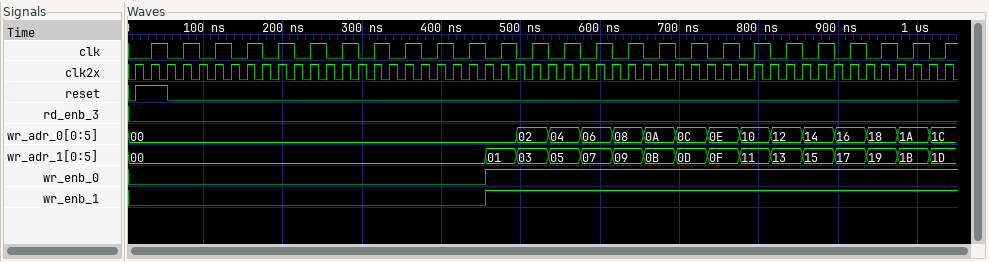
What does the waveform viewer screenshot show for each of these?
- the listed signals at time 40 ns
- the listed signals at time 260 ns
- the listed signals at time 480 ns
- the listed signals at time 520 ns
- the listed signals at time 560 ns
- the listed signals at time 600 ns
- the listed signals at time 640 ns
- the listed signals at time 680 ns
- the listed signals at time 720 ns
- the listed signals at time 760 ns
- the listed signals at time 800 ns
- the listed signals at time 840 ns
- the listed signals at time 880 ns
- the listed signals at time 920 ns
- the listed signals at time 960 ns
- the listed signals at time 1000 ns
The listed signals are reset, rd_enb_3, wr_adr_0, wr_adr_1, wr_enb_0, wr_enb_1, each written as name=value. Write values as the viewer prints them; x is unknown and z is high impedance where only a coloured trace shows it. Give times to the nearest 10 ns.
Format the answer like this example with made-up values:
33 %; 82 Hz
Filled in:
reset=1, rd_enb_3=0, wr_adr_0=00, wr_adr_1=00, wr_enb_0=0, wr_enb_1=0; reset=0, rd_enb_3=0, wr_adr_0=00, wr_adr_1=00, wr_enb_0=0, wr_enb_1=0; reset=0, rd_enb_3=0, wr_adr_0=00, wr_adr_1=01, wr_enb_0=1, wr_enb_1=1; reset=0, rd_enb_3=0, wr_adr_0=02, wr_adr_1=03, wr_enb_0=1, wr_enb_1=1; reset=0, rd_enb_3=0, wr_adr_0=04, wr_adr_1=05, wr_enb_0=1, wr_enb_1=1; reset=0, rd_enb_3=0, wr_adr_0=06, wr_adr_1=07, wr_enb_0=1, wr_enb_1=1; reset=0, rd_enb_3=0, wr_adr_0=08, wr_adr_1=09, wr_enb_0=1, wr_enb_1=1; reset=0, rd_enb_3=0, wr_adr_0=0A, wr_adr_1=0B, wr_enb_0=1, wr_enb_1=1; reset=0, rd_enb_3=0, wr_adr_0=0C, wr_adr_1=0D, wr_enb_0=1, wr_enb_1=1; reset=0, rd_enb_3=0, wr_adr_0=0E, wr_adr_1=0F, wr_enb_0=1, wr_enb_1=1; reset=0, rd_enb_3=0, wr_adr_0=10, wr_adr_1=11, wr_enb_0=1, wr_enb_1=1; reset=0, rd_enb_3=0, wr_adr_0=12, wr_adr_1=13, wr_enb_0=1, wr_enb_1=1; reset=0, rd_enb_3=0, wr_adr_0=14, wr_adr_1=15, wr_enb_0=1, wr_enb_1=1; reset=0, rd_enb_3=0, wr_adr_0=16, wr_adr_1=17, wr_enb_0=1, wr_enb_1=1; reset=0, rd_enb_3=0, wr_adr_0=18, wr_adr_1=19, wr_enb_0=1, wr_enb_1=1; reset=0, rd_enb_3=0, wr_adr_0=1A, wr_adr_1=1B, wr_enb_0=1, wr_enb_1=1
